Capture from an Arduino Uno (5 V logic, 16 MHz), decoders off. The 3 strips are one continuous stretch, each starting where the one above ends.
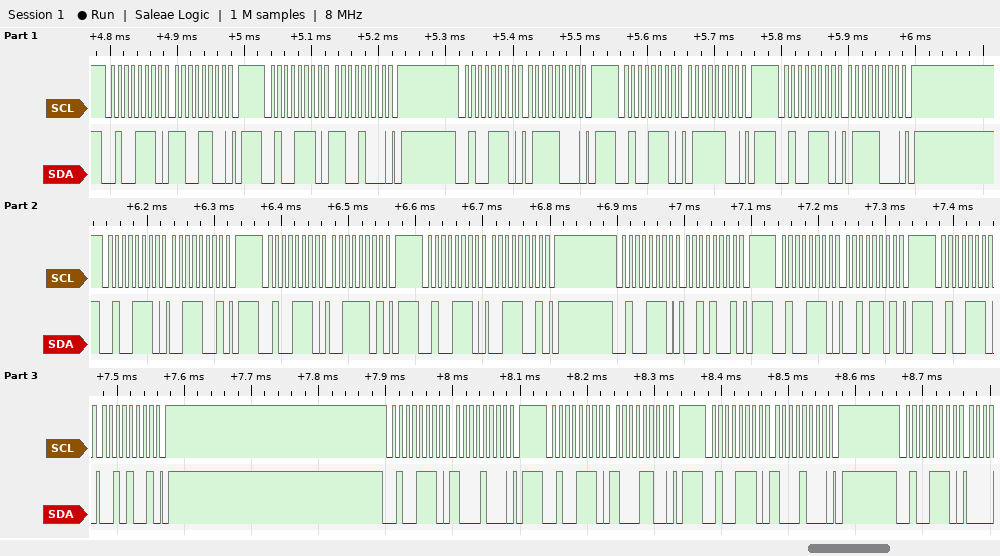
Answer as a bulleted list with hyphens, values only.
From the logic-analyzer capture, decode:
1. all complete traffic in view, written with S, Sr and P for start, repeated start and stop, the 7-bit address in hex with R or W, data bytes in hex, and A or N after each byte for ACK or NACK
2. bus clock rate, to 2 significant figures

- S 27W A CC A P S 27W A C8 A P S 27W A 78 A P S 27W A 7C A P S 27W A 78 A P S 27W A 39 A P S 27W A 3D A P S 27W A 39 A P S 27W A 29 A P S 27W A 2D A P S 27W A 29 A P S 27W A 88 A P S 27W A 8C A P S 27W A 88 A P S 27W A
- 100 kHz
